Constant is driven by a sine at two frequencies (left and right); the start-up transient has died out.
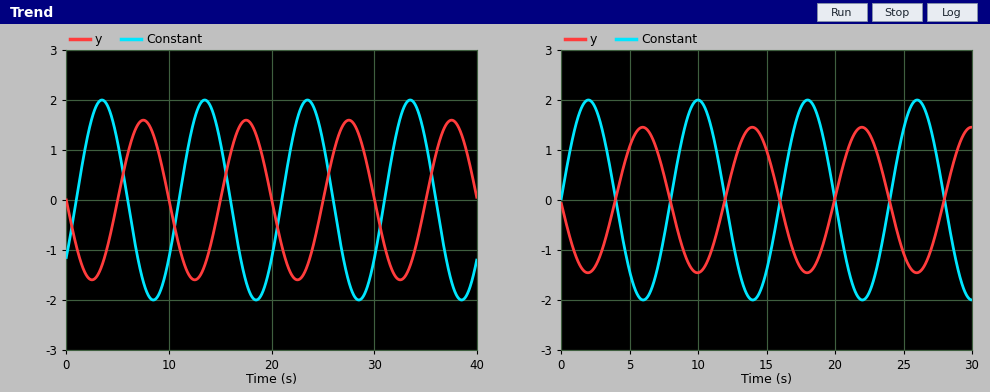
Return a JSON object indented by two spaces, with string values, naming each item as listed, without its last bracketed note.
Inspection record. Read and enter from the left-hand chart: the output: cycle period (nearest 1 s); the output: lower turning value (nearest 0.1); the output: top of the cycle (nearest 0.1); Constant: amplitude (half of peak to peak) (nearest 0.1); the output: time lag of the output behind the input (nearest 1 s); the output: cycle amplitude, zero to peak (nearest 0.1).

{
  "the output: cycle period": "10 s",
  "the output: lower turning value": "-1.6",
  "the output: top of the cycle": "1.6",
  "Constant: amplitude (half of peak to peak)": "2.0",
  "the output: time lag of the output behind the input": "4 s",
  "the output: cycle amplitude, zero to peak": "1.6"
}
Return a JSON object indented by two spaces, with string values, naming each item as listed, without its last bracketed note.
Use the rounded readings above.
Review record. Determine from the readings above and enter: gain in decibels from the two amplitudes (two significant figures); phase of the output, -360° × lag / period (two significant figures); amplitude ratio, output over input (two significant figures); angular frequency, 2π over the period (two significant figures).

{
  "gain in decibels from the two amplitudes": "-1.9 dB",
  "phase of the output, -360° × lag / period": "-140°",
  "amplitude ratio, output over input": "0.80",
  "angular frequency, 2π over the period": "0.63 rad/s"
}
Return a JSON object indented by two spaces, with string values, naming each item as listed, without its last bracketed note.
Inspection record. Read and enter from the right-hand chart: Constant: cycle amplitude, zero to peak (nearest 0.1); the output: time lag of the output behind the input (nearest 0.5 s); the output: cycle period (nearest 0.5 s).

{
  "Constant: cycle amplitude, zero to peak": "2.0",
  "the output: time lag of the output behind the input": "4.0 s",
  "the output: cycle period": "8.0 s"
}
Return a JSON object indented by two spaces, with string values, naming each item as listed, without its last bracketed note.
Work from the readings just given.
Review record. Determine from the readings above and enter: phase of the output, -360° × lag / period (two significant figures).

{
  "phase of the output, -360° × lag / period": "-180°"
}
